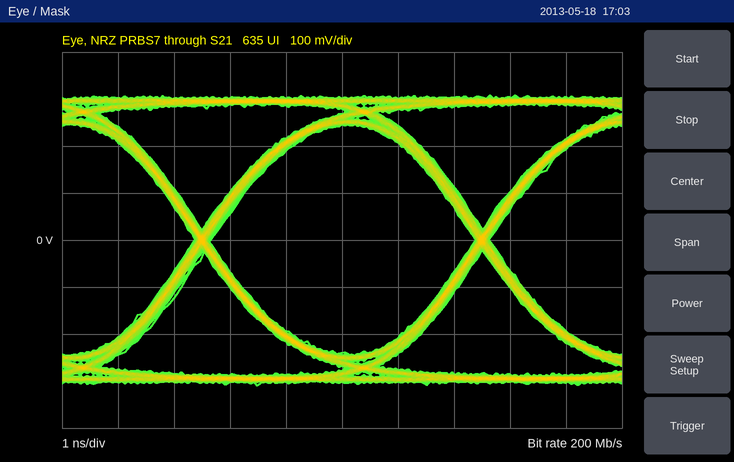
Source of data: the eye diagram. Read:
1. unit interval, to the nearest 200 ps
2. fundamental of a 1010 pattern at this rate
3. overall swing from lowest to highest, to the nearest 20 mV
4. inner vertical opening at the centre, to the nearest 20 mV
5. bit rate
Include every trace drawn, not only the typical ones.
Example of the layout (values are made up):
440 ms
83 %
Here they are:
5.0 ns
100 MHz
620 mV
480 mV
200 Mb/s
